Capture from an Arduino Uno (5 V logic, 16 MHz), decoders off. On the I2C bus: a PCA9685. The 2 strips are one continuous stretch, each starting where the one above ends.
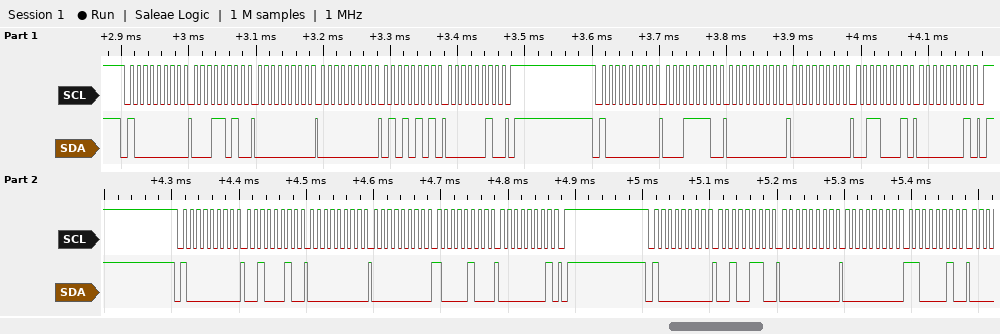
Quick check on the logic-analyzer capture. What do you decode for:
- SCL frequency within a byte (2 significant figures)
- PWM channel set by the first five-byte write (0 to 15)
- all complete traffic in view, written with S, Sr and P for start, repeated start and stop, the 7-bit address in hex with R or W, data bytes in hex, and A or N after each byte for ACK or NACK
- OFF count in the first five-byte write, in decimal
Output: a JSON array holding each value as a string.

["100 kHz", "5", "S 40W A 1A A 00 A 00 A 55 A 02 A P S 40W A 1E A 00 A 00 A 31 A 01 A P S 40W A 22 A 00 A 00 A 84 A 01 A P S 40W A 26 A 00 A 00 A C2 A", "597"]
